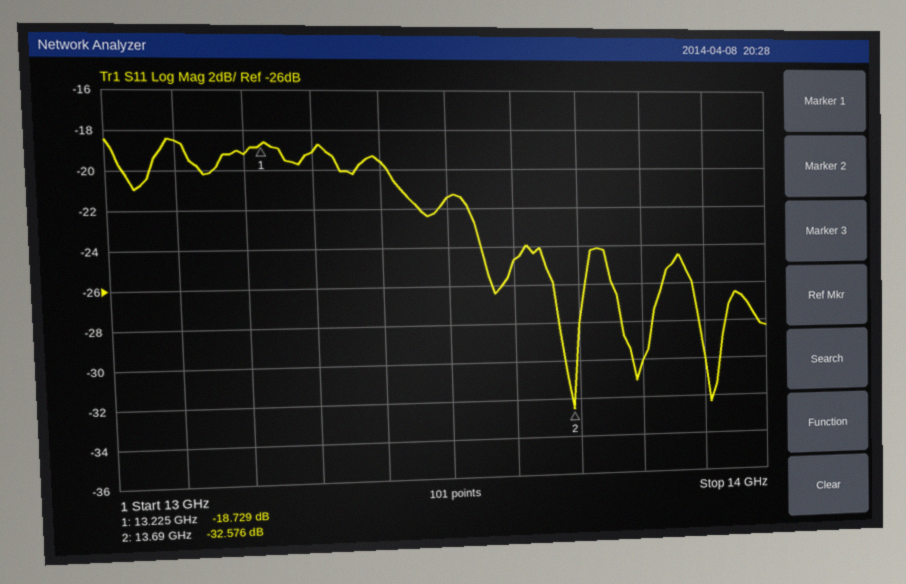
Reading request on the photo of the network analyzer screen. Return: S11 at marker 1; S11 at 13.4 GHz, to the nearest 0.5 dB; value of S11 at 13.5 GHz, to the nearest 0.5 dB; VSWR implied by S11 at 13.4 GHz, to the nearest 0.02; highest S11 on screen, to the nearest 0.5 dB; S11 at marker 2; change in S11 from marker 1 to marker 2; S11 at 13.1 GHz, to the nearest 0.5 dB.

-18.729 dB
-19.5 dB
-21.5 dB
1.24
-18.5 dB
-32.576 dB
-13.847 dB
-18.5 dB
